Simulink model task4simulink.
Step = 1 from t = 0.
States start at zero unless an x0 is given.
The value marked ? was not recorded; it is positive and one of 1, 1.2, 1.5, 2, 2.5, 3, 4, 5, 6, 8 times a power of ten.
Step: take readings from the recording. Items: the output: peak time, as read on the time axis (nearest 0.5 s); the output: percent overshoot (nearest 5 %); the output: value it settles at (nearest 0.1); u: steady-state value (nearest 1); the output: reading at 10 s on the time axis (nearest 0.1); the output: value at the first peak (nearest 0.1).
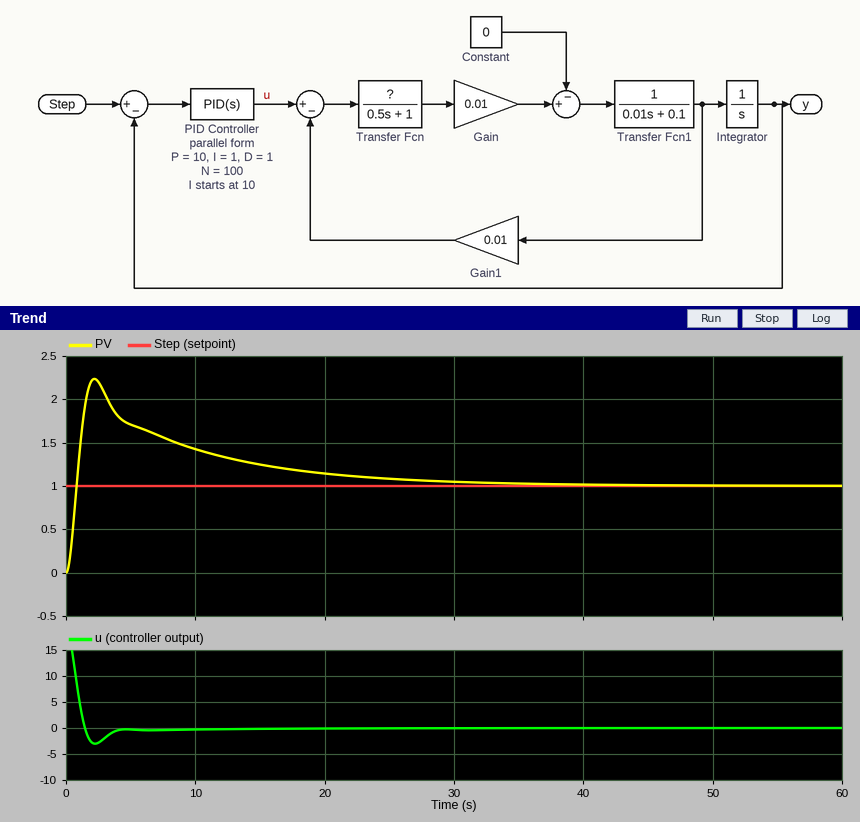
2.0 s
125 %
1.0
0
1.4
2.2
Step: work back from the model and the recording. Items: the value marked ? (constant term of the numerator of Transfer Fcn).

1.5
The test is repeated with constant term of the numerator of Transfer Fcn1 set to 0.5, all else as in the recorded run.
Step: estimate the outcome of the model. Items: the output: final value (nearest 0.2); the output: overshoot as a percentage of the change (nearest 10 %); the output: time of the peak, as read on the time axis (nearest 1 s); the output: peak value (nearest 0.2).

1.0
100 %
4 s
2.0
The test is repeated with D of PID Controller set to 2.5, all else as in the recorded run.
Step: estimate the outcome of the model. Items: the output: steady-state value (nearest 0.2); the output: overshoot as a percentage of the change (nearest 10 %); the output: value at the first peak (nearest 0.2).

1.0
110 %
2.0
